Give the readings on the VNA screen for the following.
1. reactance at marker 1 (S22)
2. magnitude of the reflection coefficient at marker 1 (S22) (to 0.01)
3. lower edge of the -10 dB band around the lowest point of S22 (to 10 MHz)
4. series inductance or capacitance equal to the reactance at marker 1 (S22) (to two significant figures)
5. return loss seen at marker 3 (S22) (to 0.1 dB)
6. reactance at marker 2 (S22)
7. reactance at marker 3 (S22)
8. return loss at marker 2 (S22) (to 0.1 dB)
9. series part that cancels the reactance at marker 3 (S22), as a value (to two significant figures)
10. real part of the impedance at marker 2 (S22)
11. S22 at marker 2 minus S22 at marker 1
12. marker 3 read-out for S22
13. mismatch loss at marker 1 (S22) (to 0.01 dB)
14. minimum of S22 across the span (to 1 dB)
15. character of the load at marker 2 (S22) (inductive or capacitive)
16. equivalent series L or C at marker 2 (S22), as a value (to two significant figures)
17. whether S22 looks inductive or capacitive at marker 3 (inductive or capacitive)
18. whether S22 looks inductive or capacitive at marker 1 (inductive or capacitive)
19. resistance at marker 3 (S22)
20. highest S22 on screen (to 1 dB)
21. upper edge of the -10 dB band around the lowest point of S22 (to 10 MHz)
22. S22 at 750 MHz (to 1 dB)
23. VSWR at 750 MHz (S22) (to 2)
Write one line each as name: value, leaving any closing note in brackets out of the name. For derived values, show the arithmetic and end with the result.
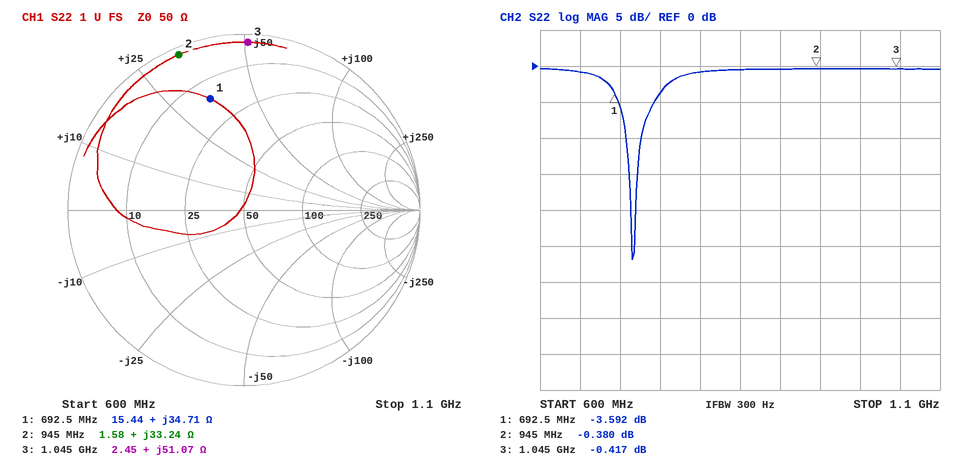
reactance at marker 1: +34.71 Ω
magnitude of the reflection coefficient at marker 1 (S22): 0.66
lower edge of the -10 dB band around the lowest point of S22: 710 MHz
series inductance or capacitance equal to the reactance at marker 1 (S22): L = 34.71 Ω/(2π × 692.5 MHz) ≈ 8.0 nH
return loss seen at marker 3 (S22): 0.4 dB
reactance at marker 2: +33.24 Ω
reactance at marker 3: +51.07 Ω
return loss at marker 2 (S22): 0.4 dB
series part that cancels the reactance at marker 3 (S22), as a value: C = 1/(2π × 1.045 GHz × 51.07 Ω) ≈ 3.0 pF
real part of the impedance at marker 2: 1.58 Ω
S22 at marker 2 minus S22 at marker 1: -0.38 − (-3.592) = 3.212 dB
marker 3 read-out for S22: -0.417 dB
mismatch loss at marker 1 (S22): −10 log10(1 − 10^(-3.592/10)) ≈ 2.50 dB
minimum of S22 across the span: -27 dB
character of the load at marker 2 (S22): inductive
equivalent series L or C at marker 2 (S22), as a value: L = 33.24 Ω/(2π × 945 MHz) ≈ 5.6 nH
whether S22 looks inductive or capacitive at marker 3: inductive
whether S22 looks inductive or capacitive at marker 1: inductive
resistance at marker 3: 2.45 Ω
highest S22 on screen: 0 dB
upper edge of the -10 dB band around the lowest point of S22: 730 MHz
S22 at 750 MHz: -4 dB
VSWR at 750 MHz (S22): |Γ| = 10^(-4/20) = 0.6310; VSWR = (1 + 0.6310)/(1 − 0.6310) ≈ 4
